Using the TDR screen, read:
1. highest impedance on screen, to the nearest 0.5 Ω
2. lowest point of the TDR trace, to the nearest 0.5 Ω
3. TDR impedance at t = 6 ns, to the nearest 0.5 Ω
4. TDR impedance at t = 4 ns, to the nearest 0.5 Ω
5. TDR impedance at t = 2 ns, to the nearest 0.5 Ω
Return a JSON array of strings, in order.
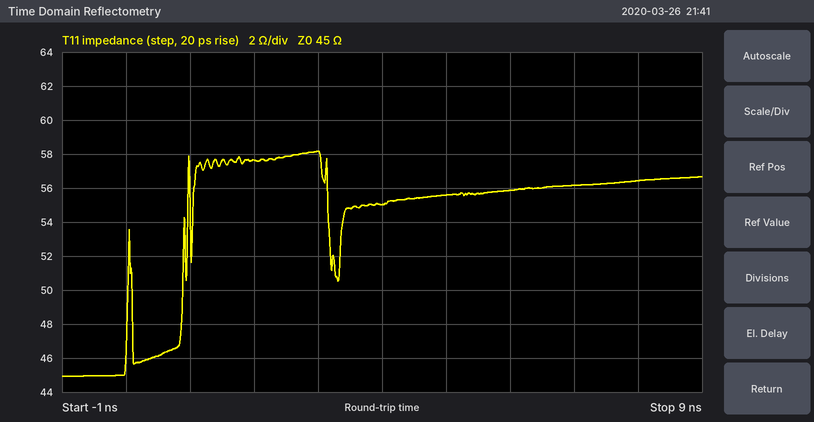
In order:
["58.0 Ω", "45.0 Ω", "56.0 Ω", "55.0 Ω", "57.5 Ω"]
